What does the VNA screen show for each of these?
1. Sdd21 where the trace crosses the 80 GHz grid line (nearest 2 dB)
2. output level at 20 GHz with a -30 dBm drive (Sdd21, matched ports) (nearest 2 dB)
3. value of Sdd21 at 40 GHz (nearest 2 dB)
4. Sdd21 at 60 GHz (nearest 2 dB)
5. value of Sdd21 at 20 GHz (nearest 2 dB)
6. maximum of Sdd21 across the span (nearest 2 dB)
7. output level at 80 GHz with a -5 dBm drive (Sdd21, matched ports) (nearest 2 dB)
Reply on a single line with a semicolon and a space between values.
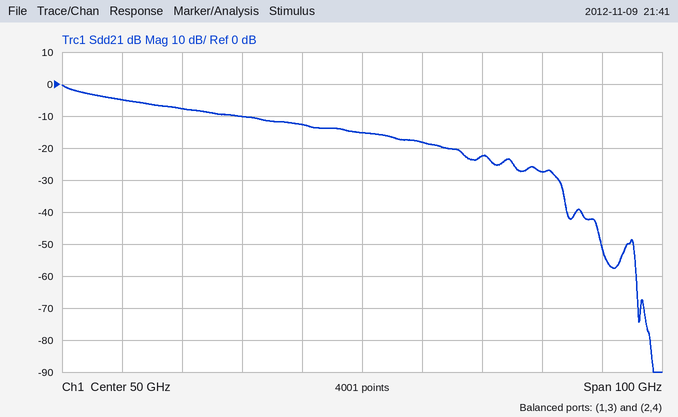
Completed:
-28 dB; -38 dBm; -12 dB; -18 dB; -8 dB; 0 dB; -32 dBm
